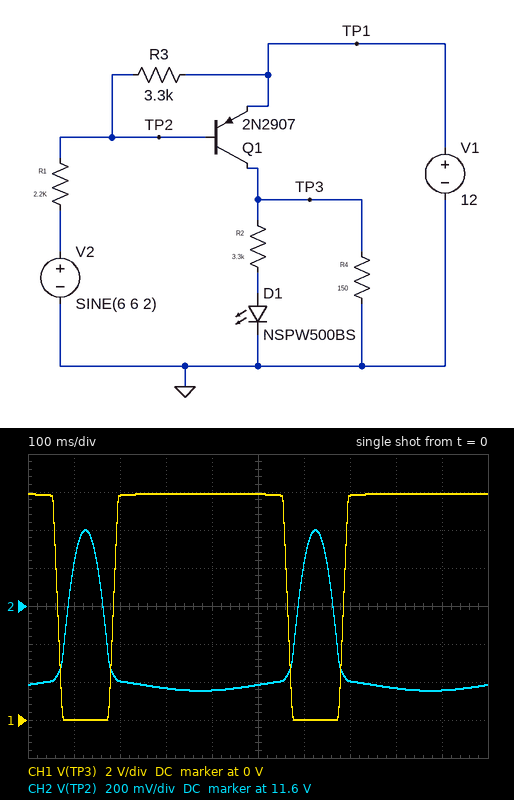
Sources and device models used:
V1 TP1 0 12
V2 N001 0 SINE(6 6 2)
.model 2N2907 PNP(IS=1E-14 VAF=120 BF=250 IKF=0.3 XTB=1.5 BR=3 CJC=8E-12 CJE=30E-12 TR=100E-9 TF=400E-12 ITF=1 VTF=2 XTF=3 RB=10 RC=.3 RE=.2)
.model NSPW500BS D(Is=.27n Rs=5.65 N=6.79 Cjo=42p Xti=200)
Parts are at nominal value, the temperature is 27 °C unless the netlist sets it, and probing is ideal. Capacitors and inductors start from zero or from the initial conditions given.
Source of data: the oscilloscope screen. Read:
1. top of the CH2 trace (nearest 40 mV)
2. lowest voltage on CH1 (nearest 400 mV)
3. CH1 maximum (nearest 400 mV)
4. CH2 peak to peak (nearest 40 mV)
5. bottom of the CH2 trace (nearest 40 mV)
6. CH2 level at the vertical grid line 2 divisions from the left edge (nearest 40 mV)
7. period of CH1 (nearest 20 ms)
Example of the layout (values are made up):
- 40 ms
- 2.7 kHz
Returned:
- 12.00 V
- 0 V
- 12.0 V
- 840 mV
- 11.16 V
- 11.20 V
- 500 ms
